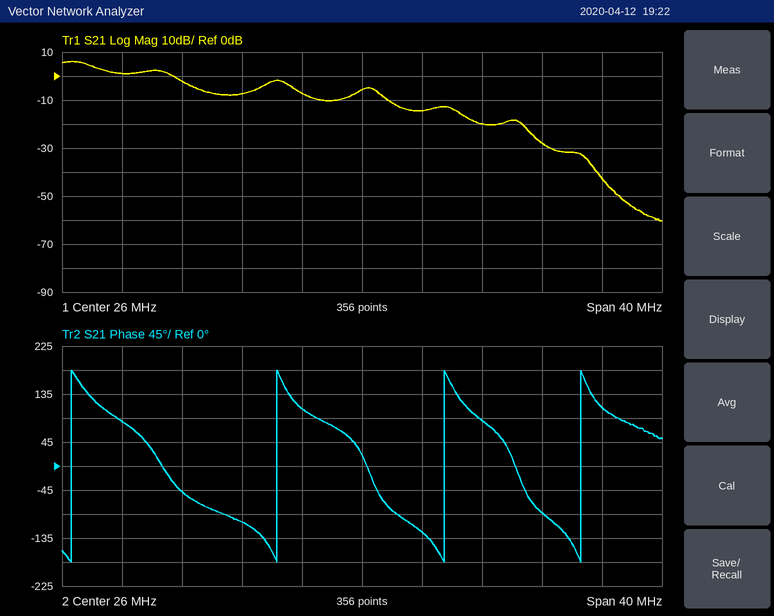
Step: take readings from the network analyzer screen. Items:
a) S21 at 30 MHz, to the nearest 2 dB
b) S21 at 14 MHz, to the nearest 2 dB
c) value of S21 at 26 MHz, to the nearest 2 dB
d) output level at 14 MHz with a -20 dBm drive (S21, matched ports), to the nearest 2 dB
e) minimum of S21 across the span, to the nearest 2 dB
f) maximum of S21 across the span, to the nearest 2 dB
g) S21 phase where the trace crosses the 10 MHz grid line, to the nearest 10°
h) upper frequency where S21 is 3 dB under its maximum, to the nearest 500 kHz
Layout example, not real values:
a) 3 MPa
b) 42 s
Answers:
a) -14 dB
b) -2 dB
c) -6 dB
d) -22 dBm
e) -60 dB
f) 6 dB
g) 80°
h) 8.5 MHz
